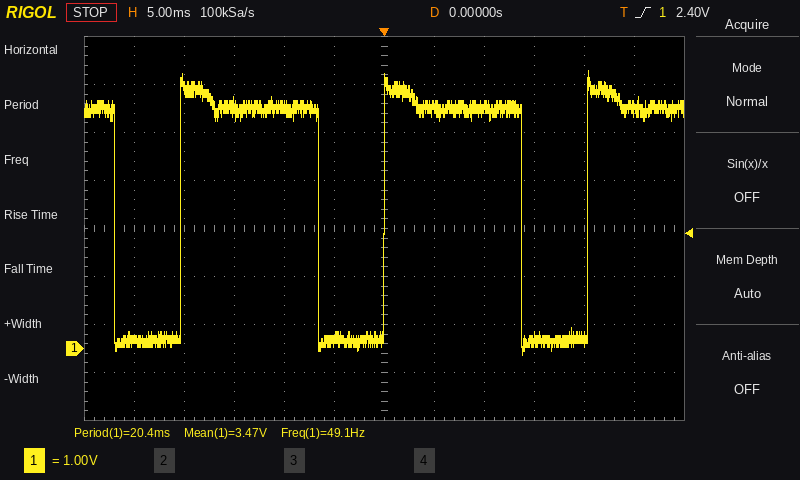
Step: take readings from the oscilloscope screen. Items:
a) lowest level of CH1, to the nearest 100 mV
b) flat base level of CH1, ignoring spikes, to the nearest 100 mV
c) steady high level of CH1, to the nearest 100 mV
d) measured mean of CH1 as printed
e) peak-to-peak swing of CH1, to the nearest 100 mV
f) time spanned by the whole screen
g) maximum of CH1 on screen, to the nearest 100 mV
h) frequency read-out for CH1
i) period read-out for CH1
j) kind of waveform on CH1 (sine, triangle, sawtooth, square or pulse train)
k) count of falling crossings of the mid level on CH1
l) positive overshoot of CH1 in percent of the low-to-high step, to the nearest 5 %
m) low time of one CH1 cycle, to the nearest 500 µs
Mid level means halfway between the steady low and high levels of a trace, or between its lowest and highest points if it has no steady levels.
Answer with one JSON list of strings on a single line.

["-100 mV", "200 mV", "5.0 V", "3.47 V", "5.9 V", "60 ms", "5.8 V", "49.1 Hz", "20.4 ms", "pulse train", "3", "15 %", "6.5 ms"]
